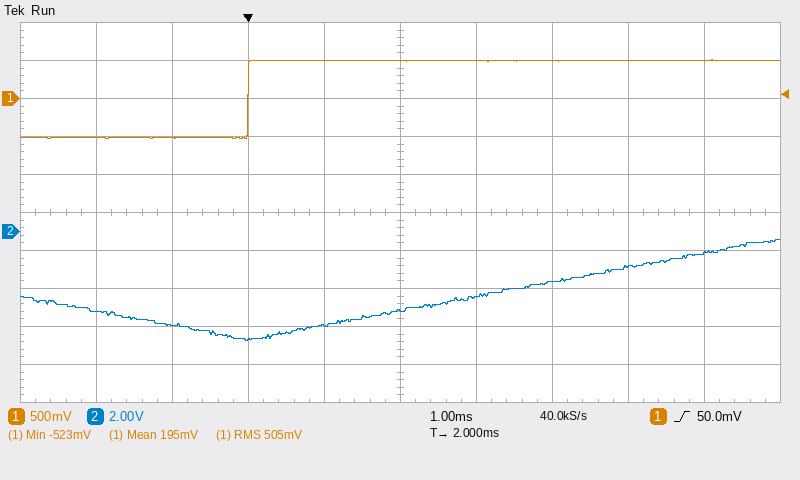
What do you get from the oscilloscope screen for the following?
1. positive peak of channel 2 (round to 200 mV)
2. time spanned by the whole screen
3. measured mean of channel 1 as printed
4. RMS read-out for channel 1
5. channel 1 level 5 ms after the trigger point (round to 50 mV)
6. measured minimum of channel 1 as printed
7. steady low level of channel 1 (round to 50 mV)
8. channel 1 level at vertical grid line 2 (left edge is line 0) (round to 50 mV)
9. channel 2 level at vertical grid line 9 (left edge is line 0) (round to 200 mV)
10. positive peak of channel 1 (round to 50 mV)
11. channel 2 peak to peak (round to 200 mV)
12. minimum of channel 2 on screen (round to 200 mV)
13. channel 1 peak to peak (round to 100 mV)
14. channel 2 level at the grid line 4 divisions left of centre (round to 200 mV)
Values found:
-400 mV
10 ms
195 mV
505 mV
500 mV
-523 mV
-500 mV
-500 mV
-1.2 V
500 mV
5.4 V
-5.8 V
1.00 V
-4.2 V
